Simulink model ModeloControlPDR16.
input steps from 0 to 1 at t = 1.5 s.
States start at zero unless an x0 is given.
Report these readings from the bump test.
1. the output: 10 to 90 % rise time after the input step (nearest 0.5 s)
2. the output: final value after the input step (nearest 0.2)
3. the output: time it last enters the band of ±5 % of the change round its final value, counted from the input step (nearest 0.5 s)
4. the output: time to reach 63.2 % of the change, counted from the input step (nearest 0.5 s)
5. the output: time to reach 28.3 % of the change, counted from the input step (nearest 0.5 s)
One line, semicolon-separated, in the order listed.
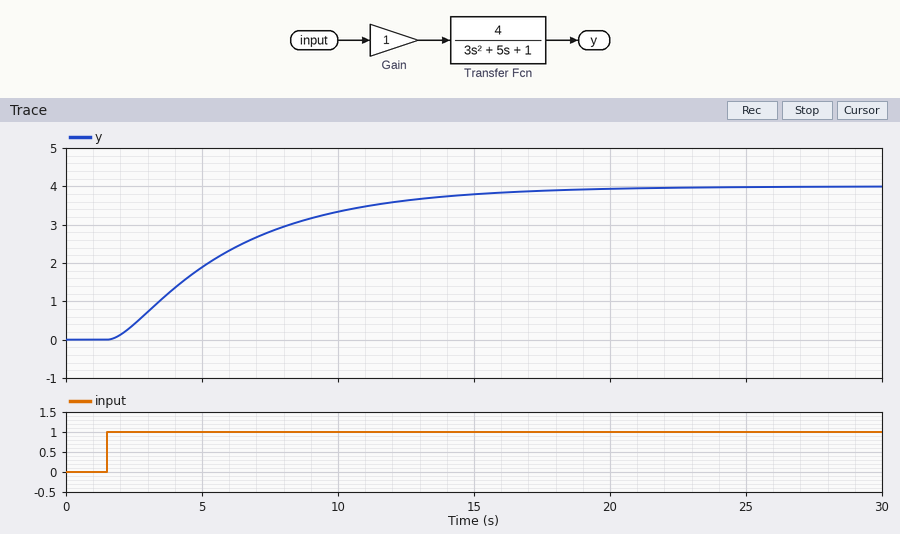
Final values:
9.5 s; 4.0; 13.5 s; 5.0 s; 2.0 s
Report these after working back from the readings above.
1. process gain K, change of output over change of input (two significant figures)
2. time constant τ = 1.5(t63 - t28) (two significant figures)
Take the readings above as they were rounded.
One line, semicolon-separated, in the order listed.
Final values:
4.0; 4.5 s
